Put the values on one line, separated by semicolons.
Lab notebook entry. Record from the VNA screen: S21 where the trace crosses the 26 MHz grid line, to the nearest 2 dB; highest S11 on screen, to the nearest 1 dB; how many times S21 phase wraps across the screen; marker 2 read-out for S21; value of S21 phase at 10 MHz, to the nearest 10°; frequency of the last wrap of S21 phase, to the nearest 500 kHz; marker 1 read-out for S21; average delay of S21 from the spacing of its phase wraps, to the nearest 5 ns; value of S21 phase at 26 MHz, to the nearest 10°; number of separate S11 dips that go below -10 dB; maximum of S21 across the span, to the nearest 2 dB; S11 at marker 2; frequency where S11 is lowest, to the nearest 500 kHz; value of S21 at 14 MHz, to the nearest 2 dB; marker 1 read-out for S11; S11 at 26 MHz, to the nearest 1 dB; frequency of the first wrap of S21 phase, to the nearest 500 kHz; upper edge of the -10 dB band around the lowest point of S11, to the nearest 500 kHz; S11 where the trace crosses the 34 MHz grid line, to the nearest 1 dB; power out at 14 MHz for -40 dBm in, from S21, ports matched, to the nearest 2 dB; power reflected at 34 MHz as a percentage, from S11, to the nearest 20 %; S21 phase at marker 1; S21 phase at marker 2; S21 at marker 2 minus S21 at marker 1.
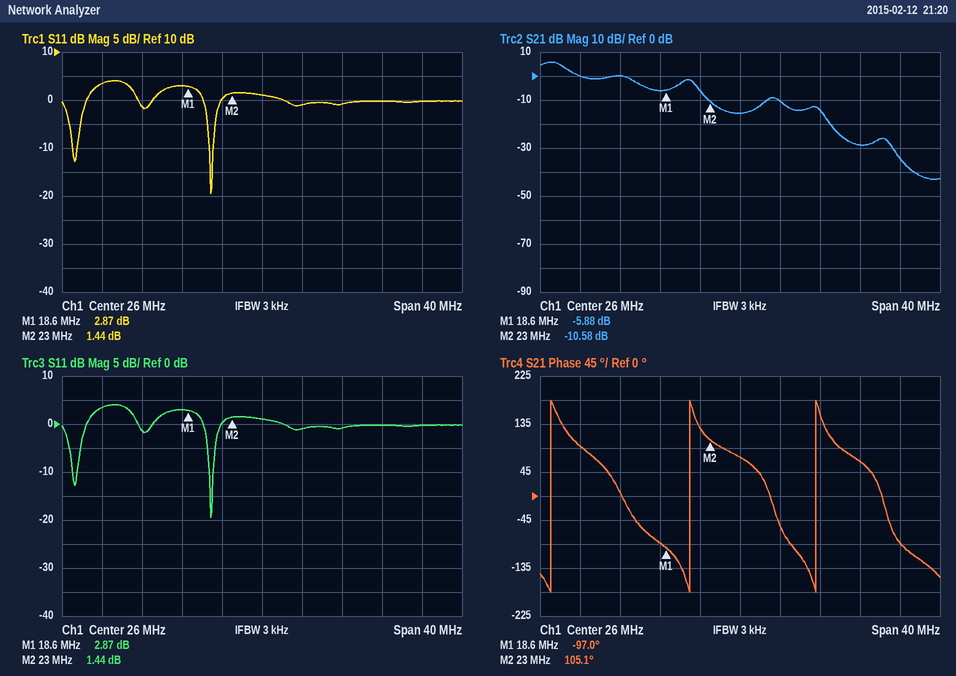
-16 dB; 4 dB; 3; -10.58 dB; 90°; 33.5 MHz; -5.88 dB; 75 ns; 70°; 2; 6 dB; 1.44 dB; 21.0 MHz; 0 dB; 2.87 dB; 1 dB; 7.0 MHz; 21.0 MHz; -1 dB; -40 dBm; 80 %; -97.0°; 105.1°; -4.70 dB
